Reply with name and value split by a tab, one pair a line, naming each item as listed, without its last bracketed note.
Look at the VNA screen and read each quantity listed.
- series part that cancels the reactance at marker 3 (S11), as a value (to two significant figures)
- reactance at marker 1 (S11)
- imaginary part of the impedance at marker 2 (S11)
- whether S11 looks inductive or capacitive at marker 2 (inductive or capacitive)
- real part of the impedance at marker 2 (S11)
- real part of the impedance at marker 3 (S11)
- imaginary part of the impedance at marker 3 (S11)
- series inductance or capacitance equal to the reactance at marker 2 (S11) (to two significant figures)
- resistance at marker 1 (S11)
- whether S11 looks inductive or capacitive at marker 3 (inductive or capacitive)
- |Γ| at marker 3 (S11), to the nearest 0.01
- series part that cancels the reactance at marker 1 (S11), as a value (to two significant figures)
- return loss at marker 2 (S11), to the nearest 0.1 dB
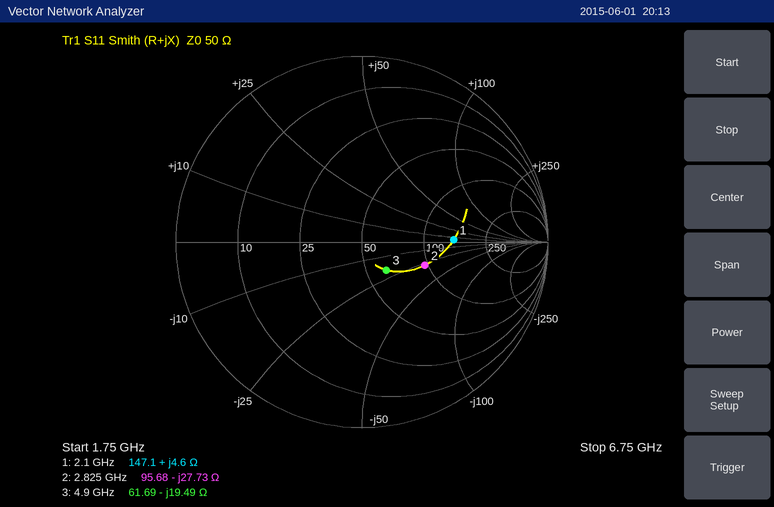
series part that cancels the reactance at marker 3 (S11), as a value	630 pH
reactance at marker 1	+4.6 Ω
imaginary part of the impedance at marker 2	-27.73 Ω
whether S11 looks inductive or capacitive at marker 2	capacitive
real part of the impedance at marker 2	95.68 Ω
real part of the impedance at marker 3	61.69 Ω
imaginary part of the impedance at marker 3	-19.49 Ω
series inductance or capacitance equal to the reactance at marker 2 (S11)	2.0 pF
resistance at marker 1	147.1 Ω
whether S11 looks inductive or capacitive at marker 3	capacitive
|Γ| at marker 3 (S11), to the nearest 0.01	0.20
series part that cancels the reactance at marker 1 (S11), as a value	16 pF
return loss at marker 2 (S11), to the nearest 0.1 dB	8.9 dB
